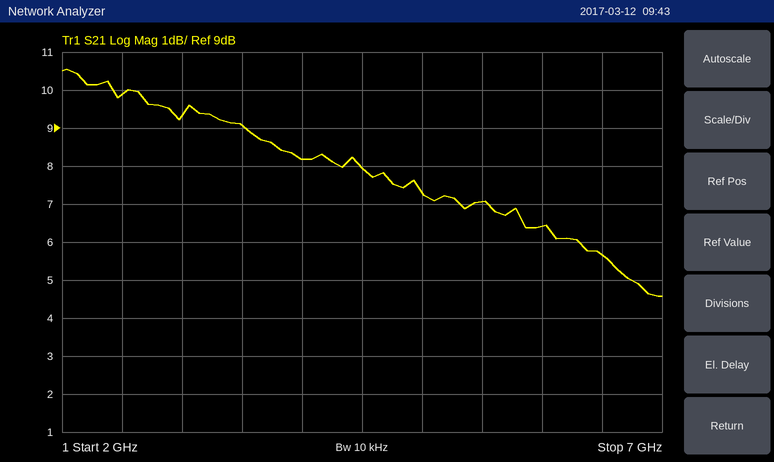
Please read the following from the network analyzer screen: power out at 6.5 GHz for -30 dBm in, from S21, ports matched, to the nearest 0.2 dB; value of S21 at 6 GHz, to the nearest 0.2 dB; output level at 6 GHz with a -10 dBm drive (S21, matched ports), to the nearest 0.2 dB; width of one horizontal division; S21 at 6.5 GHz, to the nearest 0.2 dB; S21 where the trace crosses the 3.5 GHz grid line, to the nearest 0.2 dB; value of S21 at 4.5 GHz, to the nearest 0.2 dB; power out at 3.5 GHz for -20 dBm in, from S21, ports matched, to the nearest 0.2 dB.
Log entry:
-24.4 dBm
6.4 dB
-3.6 dBm
500 MHz
5.6 dB
9.0 dB
8.0 dB
-11.0 dBm
